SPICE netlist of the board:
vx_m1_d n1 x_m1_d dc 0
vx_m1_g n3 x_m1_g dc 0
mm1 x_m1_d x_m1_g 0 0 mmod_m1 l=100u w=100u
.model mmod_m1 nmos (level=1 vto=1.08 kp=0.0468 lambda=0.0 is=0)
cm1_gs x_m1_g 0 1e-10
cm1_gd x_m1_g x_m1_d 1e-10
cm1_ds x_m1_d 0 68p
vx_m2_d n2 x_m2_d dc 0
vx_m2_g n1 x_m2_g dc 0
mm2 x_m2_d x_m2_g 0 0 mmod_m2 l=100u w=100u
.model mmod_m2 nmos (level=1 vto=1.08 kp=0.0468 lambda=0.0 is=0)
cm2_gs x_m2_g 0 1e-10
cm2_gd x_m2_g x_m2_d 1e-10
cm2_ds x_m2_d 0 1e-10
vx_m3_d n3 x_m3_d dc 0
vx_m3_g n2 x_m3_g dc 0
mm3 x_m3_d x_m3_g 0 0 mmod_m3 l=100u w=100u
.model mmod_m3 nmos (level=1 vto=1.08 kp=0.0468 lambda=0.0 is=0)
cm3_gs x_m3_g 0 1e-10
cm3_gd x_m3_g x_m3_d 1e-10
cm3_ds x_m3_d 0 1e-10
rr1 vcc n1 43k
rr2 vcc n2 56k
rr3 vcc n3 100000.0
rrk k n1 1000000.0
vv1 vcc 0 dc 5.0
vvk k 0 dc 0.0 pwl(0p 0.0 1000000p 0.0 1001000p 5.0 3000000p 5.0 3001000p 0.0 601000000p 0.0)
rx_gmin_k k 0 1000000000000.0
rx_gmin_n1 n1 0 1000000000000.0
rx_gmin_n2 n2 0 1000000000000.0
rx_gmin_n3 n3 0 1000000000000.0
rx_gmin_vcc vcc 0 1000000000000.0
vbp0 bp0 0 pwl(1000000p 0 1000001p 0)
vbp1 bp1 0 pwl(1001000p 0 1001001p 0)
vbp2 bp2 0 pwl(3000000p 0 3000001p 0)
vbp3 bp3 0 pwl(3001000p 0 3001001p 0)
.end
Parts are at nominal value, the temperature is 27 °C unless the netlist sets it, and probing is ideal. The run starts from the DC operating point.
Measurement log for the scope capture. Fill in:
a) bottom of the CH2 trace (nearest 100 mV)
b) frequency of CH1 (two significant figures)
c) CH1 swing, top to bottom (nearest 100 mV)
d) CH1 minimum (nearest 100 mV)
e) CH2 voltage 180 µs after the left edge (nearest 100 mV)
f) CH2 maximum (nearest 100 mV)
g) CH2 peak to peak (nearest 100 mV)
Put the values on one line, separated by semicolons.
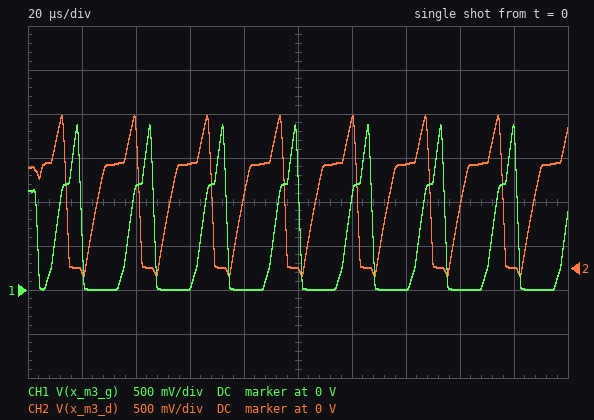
-100 mV; 37 kHz; 1.9 V; 0 V; 0 V; 1.7 V; 1.8 V
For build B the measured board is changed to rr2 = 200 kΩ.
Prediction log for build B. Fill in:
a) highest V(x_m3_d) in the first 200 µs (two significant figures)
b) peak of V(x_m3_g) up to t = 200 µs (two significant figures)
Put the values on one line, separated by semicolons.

2.6 V; 1.4 V
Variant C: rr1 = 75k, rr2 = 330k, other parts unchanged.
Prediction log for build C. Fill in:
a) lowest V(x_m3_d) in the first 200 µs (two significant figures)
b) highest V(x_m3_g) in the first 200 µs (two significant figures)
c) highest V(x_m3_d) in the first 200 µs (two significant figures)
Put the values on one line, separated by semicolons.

2.1 mV; 1.4 V; 3.1 V
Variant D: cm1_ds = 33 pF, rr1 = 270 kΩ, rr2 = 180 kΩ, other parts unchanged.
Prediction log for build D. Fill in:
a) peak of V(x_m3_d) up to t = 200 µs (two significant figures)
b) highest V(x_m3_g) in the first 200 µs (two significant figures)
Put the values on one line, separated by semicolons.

2.5 V; 2.2 V
